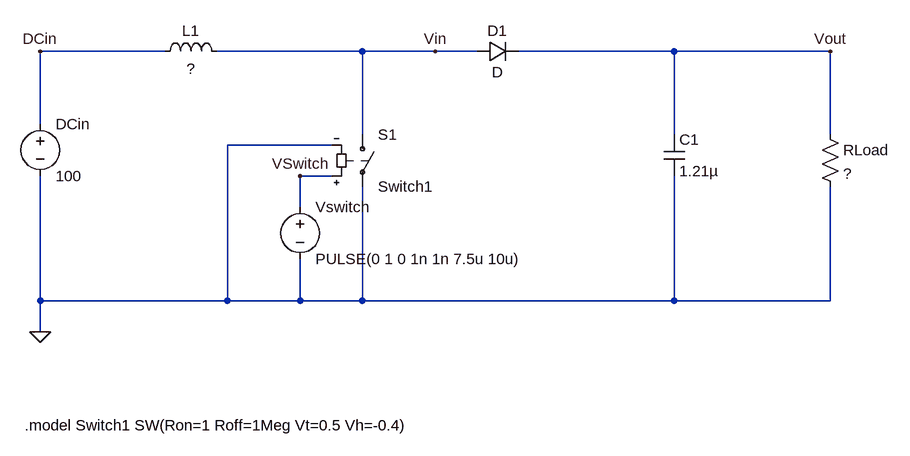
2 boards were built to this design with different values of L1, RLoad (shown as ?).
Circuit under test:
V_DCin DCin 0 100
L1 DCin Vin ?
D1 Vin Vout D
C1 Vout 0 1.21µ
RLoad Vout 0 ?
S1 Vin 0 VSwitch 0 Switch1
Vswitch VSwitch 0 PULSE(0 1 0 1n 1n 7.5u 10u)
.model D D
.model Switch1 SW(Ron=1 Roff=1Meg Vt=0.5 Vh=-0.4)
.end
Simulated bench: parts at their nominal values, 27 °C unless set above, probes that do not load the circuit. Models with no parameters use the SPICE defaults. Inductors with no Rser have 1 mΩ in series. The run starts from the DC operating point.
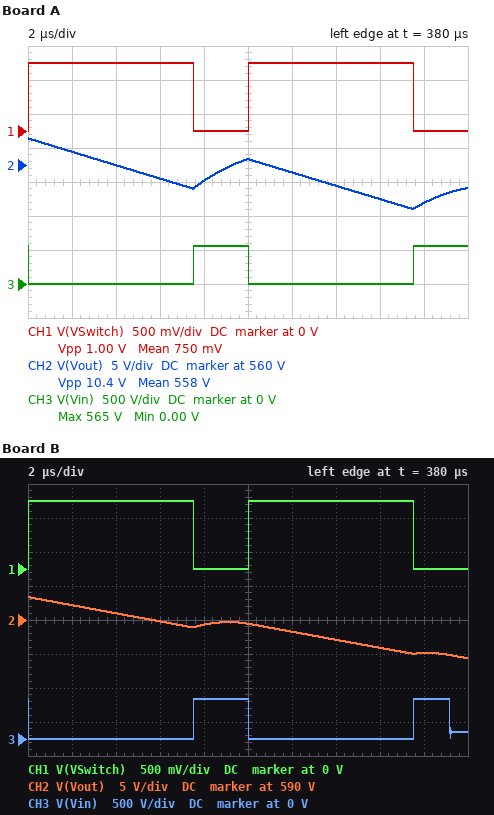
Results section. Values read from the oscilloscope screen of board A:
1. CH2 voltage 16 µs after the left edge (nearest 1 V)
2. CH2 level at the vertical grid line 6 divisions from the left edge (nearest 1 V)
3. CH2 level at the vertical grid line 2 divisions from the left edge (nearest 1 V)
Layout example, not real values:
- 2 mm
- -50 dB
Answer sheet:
- 555 V
- 559 V
- 560 V
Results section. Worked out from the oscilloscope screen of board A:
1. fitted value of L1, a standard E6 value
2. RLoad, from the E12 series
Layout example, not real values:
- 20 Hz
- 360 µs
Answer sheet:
- 680 µH
- 470 Ω
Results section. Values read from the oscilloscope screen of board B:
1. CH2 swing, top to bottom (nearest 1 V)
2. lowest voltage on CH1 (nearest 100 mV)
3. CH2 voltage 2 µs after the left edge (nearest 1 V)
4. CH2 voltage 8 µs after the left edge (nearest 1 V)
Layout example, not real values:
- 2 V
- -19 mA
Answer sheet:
- 9 V
- 0 V
- 592 V
- 589 V
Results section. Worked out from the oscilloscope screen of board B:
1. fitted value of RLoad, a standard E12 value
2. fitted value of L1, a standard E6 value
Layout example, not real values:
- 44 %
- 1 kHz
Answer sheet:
- 820 Ω
- 680 µH
